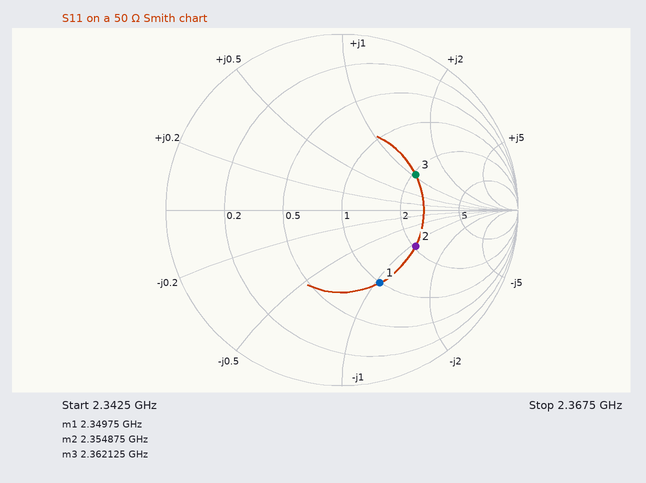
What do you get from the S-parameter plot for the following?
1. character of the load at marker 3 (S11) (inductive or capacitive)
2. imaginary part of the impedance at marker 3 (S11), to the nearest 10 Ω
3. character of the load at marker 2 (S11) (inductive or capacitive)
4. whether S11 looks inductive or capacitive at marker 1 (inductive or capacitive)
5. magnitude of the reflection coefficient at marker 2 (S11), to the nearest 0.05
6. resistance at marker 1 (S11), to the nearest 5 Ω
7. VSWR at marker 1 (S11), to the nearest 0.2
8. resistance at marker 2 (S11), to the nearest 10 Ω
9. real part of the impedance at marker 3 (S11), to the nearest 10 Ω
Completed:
inductive
+50 Ω
capacitive
capacitive
0.45
50 Ω
2.8
100 Ω
100 Ω
